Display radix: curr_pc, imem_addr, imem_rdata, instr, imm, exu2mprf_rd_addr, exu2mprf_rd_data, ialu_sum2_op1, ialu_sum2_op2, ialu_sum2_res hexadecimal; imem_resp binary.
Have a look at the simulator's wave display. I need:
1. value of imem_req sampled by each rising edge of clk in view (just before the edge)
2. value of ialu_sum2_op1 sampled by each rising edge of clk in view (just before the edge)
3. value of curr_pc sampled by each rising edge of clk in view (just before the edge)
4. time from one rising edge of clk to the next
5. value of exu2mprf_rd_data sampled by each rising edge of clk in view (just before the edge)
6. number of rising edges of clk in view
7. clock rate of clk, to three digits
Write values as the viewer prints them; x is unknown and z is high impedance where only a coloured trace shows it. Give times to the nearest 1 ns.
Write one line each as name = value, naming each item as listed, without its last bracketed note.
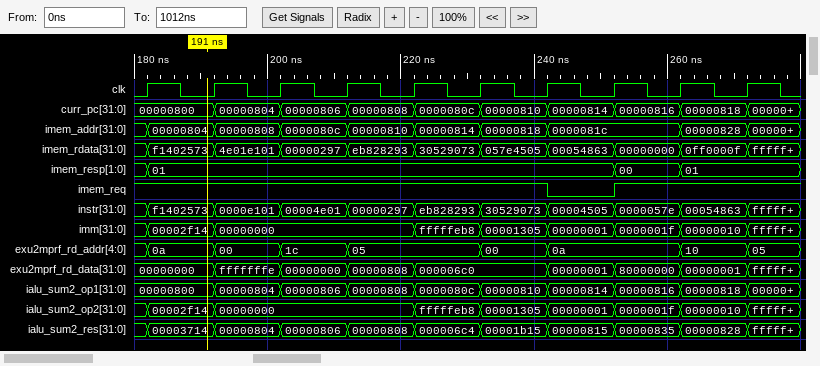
value of imem_req sampled by each rising edge of clk in view = 1 1 1 1 1 1 1 0 1 1
value of ialu_sum2_op1 sampled by each rising edge of clk in view = 00000800, 00000800, 00000804, 00000806, 00000808, 0000080c, 00000810, 00000814, 00000816, 00000818
value of curr_pc sampled by each rising edge of clk in view = 00000800, 00000800, 00000804, 00000806, 00000808, 0000080c, 00000810, 00000814, 00000816, 00000818
time from one rising edge of clk to the next = 10 ns
value of exu2mprf_rd_data sampled by each rising edge of clk in view = 00000000, 00000000, fffffffe, 00000000, 00000808, 000006c0, 000006c0, 00000001, 80000000, 00000001
number of rising edges of clk in view = 10
clock rate of clk, to three digits = 100 MHz
